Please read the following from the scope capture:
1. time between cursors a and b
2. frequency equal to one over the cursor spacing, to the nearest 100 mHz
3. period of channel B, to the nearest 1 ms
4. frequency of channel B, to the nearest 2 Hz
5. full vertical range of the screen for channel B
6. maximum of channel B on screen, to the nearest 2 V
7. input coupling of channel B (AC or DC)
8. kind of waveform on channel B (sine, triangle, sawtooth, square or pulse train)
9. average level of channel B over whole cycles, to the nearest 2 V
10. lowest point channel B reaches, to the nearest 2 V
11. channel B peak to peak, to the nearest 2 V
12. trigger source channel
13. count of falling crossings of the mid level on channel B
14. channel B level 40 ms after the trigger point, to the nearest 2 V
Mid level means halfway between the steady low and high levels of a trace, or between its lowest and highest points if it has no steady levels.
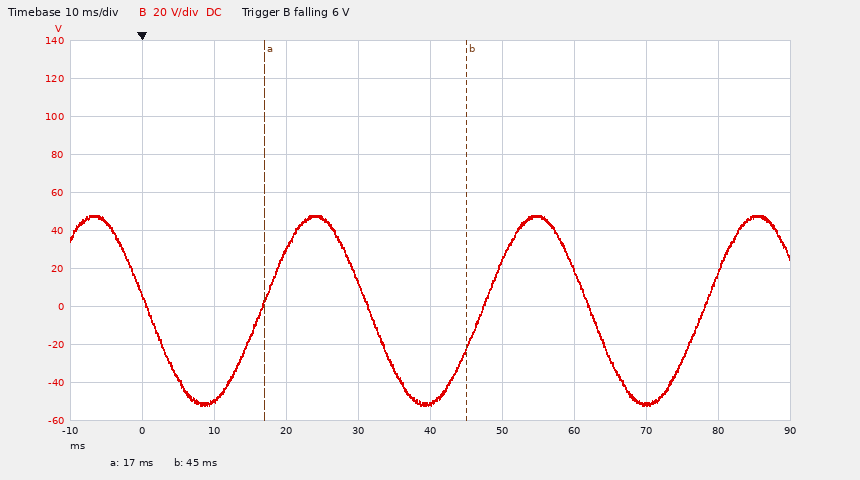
28 ms
35.7 Hz
31 ms
32 Hz
200 V
48 V
DC
sine
-2 V
-52 V
100 V
channel B
3
-50 V
